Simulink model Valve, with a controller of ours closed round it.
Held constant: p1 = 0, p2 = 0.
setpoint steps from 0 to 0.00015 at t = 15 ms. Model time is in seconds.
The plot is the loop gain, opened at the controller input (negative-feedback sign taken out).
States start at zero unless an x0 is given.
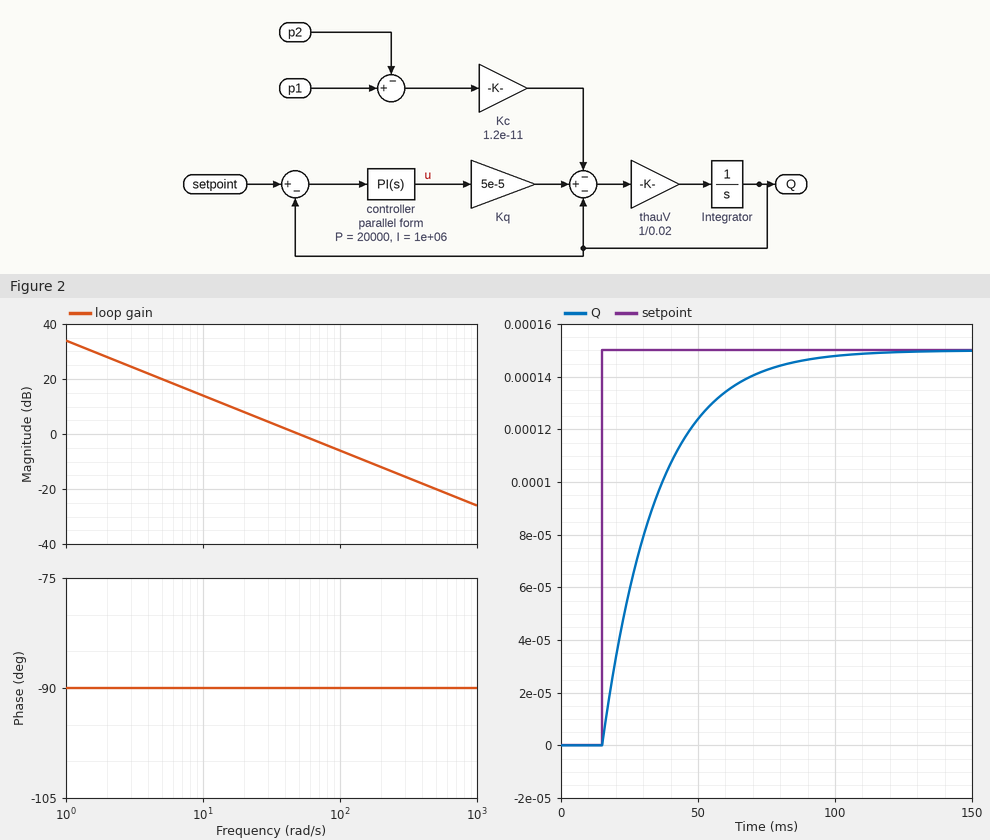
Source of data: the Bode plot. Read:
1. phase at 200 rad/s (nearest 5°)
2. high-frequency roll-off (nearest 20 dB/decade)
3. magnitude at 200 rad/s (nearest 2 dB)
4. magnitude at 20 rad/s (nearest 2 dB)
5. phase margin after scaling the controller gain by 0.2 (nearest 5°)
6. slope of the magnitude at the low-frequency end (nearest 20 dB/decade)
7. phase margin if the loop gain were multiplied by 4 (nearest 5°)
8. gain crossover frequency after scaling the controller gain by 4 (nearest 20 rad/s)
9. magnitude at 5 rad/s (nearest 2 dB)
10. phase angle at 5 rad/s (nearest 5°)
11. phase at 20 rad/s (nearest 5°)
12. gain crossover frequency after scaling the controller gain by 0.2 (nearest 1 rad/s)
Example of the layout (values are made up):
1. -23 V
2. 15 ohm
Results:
1. -90°
2. -20 dB/decade
3. -12 dB
4. 8 dB
5. 90°
6. -20 dB/decade
7. 90°
8. 200 rad/s
9. 20 dB
10. -90°
11. -90°
12. 10 rad/s
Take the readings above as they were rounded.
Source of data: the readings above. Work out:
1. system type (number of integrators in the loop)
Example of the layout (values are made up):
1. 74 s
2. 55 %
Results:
1. 1
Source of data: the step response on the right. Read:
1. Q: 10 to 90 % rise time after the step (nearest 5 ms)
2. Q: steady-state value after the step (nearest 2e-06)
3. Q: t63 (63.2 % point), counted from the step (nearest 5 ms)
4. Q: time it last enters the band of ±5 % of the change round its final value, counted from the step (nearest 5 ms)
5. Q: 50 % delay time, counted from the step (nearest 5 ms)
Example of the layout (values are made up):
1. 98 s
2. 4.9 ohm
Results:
1. 45 ms
2. 0.000150
3. 20 ms
4. 60 ms
5. 15 ms
